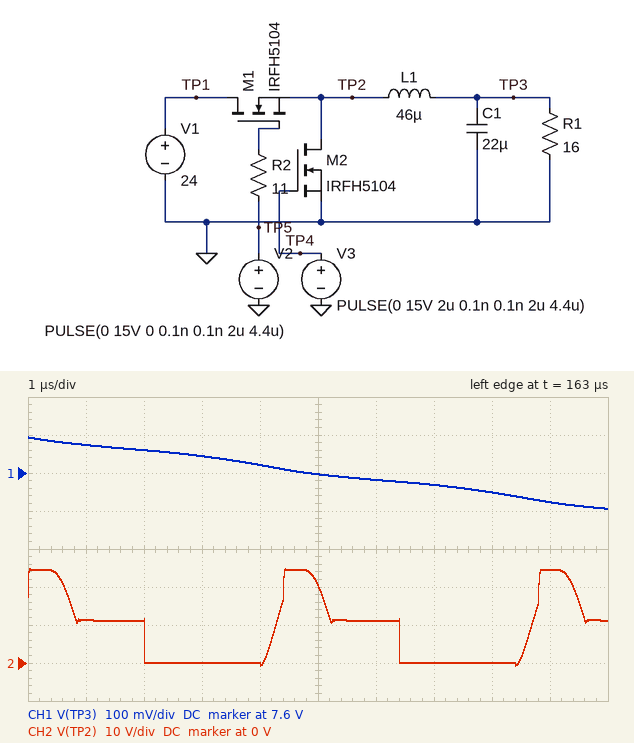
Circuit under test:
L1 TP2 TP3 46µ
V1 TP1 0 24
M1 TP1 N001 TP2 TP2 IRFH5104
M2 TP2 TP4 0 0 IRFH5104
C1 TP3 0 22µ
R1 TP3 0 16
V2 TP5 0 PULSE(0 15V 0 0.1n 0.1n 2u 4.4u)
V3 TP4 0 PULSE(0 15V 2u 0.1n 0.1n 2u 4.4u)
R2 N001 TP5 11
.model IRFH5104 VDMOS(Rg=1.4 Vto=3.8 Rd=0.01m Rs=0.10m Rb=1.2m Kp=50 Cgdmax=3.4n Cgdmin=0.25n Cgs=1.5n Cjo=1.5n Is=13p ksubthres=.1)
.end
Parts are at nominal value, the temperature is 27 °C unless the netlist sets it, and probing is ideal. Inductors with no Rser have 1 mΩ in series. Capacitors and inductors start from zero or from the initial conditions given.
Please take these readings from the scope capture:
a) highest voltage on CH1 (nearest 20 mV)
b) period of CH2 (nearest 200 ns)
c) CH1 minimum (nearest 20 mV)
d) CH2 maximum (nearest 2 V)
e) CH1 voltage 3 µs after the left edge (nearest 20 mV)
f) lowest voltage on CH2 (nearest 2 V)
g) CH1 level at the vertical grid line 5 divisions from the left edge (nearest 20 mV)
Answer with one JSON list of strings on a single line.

["7.70 V", "4.4 µs", "7.50 V", "24 V", "7.64 V", "0 V", "7.60 V"]
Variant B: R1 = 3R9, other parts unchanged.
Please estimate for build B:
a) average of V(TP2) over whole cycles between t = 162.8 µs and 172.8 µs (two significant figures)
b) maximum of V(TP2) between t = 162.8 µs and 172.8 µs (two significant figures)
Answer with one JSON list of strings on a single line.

["5.0 V", "12 V"]
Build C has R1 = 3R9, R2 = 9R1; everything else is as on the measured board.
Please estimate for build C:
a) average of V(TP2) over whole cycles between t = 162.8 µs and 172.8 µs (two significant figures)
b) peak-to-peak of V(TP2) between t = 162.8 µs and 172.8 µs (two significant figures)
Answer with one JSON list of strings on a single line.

["5.0 V", "12 V"]
